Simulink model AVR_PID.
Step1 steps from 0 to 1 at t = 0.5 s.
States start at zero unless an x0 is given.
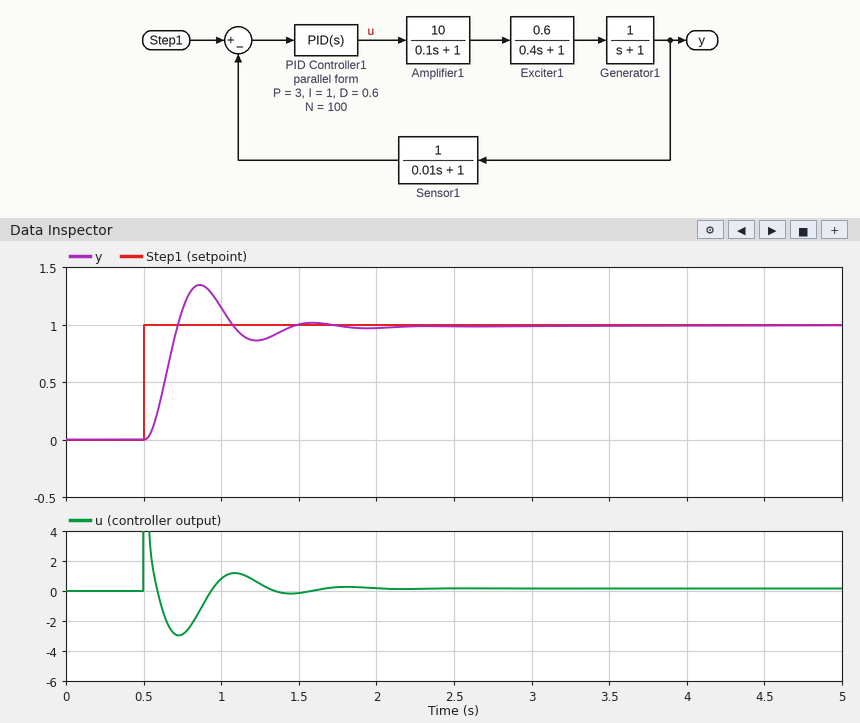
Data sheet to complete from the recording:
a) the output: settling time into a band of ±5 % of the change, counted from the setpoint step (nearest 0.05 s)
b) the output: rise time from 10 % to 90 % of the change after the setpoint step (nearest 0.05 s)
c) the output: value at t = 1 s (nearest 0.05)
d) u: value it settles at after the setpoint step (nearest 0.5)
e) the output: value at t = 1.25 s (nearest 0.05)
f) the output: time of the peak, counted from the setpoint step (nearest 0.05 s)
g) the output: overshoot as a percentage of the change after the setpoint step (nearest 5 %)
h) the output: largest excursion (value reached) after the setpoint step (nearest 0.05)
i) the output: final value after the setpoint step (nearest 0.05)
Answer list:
0.90 s
0.15 s
1.15
0.0
0.85
0.35 s
35 %
1.35
1.00
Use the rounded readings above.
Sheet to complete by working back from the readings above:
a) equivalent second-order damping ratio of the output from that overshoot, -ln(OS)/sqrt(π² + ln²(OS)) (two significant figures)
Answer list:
0.32
